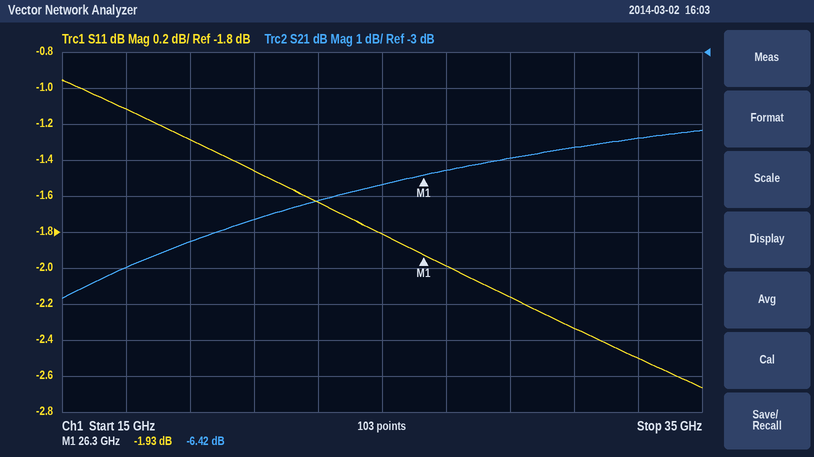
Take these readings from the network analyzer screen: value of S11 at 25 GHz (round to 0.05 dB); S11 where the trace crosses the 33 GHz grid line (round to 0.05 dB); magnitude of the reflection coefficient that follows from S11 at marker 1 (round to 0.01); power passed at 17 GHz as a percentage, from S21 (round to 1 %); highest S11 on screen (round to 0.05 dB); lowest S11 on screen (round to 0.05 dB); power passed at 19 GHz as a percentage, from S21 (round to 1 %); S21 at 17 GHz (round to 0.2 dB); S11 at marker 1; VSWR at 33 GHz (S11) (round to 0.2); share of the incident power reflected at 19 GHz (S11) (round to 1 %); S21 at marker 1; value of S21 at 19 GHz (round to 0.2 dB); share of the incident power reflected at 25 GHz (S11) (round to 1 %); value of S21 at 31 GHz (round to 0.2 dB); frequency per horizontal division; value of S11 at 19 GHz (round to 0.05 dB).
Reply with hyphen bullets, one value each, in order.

- -1.80 dB
- -2.50 dB
- 0.80
- 13 %
- -0.95 dB
- -2.65 dB
- 15 %
- -9.0 dB
- -1.93 dB
- 7.0
- 74 %
- -6.42 dB
- -8.2 dB
- 66 %
- -5.6 dB
- 2 GHz
- -1.30 dB
